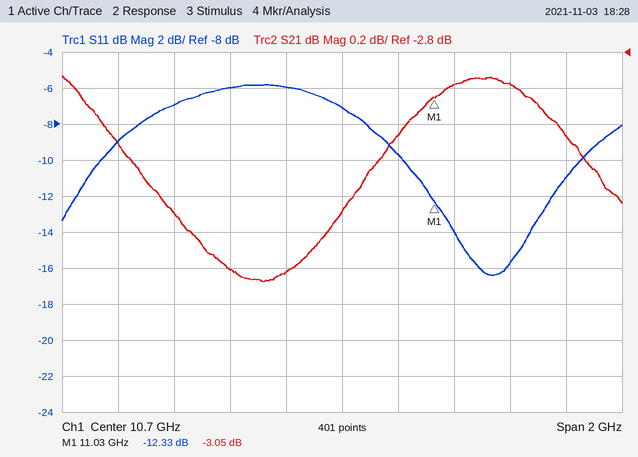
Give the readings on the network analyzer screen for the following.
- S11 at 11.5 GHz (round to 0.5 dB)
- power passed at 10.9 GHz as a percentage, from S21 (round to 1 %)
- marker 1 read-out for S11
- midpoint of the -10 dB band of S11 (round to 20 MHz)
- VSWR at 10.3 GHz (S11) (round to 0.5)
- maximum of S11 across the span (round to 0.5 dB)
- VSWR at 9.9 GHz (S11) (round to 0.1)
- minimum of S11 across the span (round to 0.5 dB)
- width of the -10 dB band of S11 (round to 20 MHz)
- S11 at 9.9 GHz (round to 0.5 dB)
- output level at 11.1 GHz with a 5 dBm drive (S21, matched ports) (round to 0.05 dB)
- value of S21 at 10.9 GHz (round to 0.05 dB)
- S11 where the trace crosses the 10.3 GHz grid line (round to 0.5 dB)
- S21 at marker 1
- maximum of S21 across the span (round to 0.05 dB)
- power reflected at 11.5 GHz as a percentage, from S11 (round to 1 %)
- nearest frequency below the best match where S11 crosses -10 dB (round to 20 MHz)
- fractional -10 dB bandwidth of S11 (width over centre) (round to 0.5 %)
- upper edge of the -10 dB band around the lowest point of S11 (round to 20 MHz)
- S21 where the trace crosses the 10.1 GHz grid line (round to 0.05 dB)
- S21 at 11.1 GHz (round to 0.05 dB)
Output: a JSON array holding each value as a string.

["-11.0 dB", "47 %", "-12.33 dB", "11.24 GHz", "3.0", "-6.0 dB", "2.1", "-16.5 dB", "640 MHz", "-9.0 dB", "2.00 dBm", "-3.25 dB", "-6.0 dB", "-3.05 dB", "-2.95 dB", "8 %", "10.92 GHz", "5.5 %", "11.56 GHz", "-3.70 dB", "-3.00 dB"]
